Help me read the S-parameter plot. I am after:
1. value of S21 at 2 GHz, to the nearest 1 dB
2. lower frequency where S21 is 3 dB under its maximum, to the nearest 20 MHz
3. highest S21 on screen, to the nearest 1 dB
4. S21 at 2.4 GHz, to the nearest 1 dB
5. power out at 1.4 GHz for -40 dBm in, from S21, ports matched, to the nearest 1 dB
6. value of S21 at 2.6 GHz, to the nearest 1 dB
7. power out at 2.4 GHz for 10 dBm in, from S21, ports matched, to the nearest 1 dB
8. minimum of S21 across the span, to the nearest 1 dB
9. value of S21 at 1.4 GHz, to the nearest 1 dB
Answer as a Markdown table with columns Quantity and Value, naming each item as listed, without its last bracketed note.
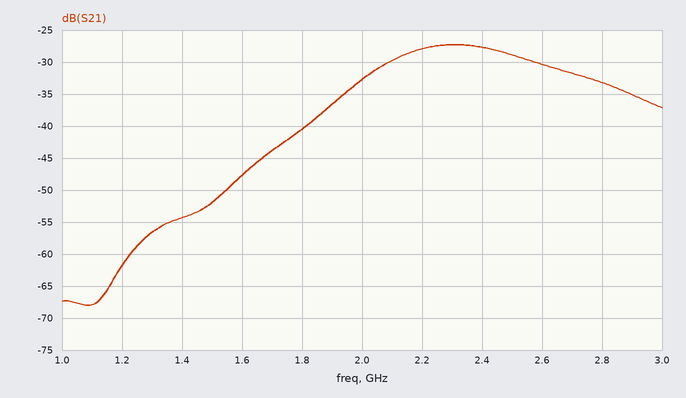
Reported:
| Quantity | Value |
|---|---|
| value of S21 at 2 GHz, to the nearest 1 dB | -33 dB |
| lower frequency where S21 is 3 dB under its maximum, to the nearest 20 MHz | 2.08 GHz |
| highest S21 on screen, to the nearest 1 dB | -27 dB |
| S21 at 2.4 GHz, to the nearest 1 dB | -28 dB |
| power out at 1.4 GHz for -40 dBm in, from S21, ports matched, to the nearest 1 dB | -94 dBm |
| value of S21 at 2.6 GHz, to the nearest 1 dB | -30 dB |
| power out at 2.4 GHz for 10 dBm in, from S21, ports matched, to the nearest 1 dB | -18 dBm |
| minimum of S21 across the span, to the nearest 1 dB | -68 dB |
| value of S21 at 1.4 GHz, to the nearest 1 dB | -54 dB |
